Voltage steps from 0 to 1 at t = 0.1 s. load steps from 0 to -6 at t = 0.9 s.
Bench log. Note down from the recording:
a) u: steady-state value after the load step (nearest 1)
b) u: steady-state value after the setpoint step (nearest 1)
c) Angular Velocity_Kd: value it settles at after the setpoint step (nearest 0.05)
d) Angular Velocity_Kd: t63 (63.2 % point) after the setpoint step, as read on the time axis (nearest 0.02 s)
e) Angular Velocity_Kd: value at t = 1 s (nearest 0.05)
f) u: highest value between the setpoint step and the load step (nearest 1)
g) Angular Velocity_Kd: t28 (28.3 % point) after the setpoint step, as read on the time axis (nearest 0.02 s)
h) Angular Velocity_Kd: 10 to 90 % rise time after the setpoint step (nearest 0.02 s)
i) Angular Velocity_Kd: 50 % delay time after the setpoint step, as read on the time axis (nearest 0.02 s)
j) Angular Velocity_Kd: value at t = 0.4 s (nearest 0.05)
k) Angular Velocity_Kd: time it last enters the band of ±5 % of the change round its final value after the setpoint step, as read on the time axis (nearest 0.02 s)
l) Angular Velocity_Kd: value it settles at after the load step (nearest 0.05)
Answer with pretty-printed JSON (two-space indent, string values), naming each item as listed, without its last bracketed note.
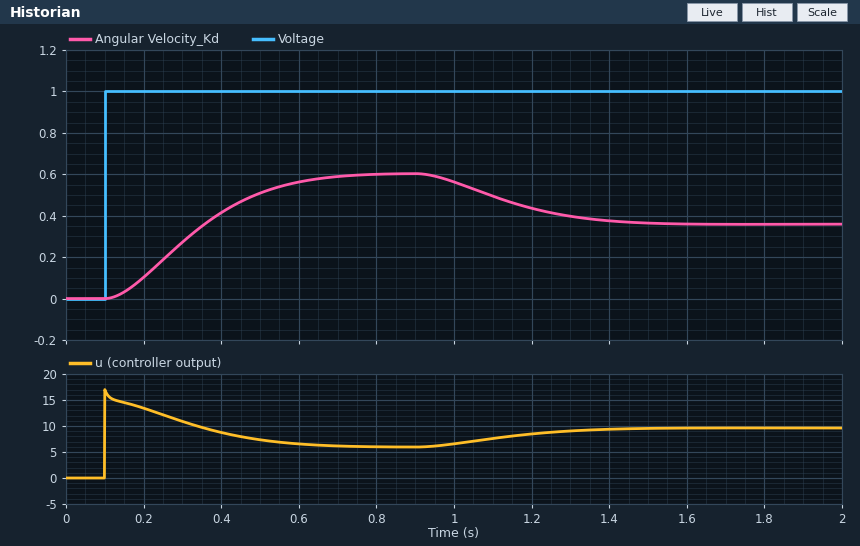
{
  "u: steady-state value after the load step": "10",
  "u: steady-state value after the setpoint step": "6",
  "Angular Velocity_Kd: value it settles at after the setpoint step": "0.60",
  "Angular Velocity_Kd: t63 (63.2 % point) after the setpoint step, as read on the time axis": "0.38 s",
  "Angular Velocity_Kd: value at t = 1 s": "0.55",
  "u: highest value between the setpoint step and the load step": "17",
  "Angular Velocity_Kd: t28 (28.3 % point) after the setpoint step, as read on the time axis": "0.24 s",
  "Angular Velocity_Kd: 10 to 90 % rise time after the setpoint step": "0.38 s",
  "Angular Velocity_Kd: 50 % delay time after the setpoint step, as read on the time axis": "0.32 s",
  "Angular Velocity_Kd: value at t = 0.4 s": "0.40",
  "Angular Velocity_Kd: time it last enters the band of ±5 % of the change round its final value after the setpoint step, as read on the time axis": "0.62 s",
  "Angular Velocity_Kd: value it settles at after the load step": "0.35"
}
